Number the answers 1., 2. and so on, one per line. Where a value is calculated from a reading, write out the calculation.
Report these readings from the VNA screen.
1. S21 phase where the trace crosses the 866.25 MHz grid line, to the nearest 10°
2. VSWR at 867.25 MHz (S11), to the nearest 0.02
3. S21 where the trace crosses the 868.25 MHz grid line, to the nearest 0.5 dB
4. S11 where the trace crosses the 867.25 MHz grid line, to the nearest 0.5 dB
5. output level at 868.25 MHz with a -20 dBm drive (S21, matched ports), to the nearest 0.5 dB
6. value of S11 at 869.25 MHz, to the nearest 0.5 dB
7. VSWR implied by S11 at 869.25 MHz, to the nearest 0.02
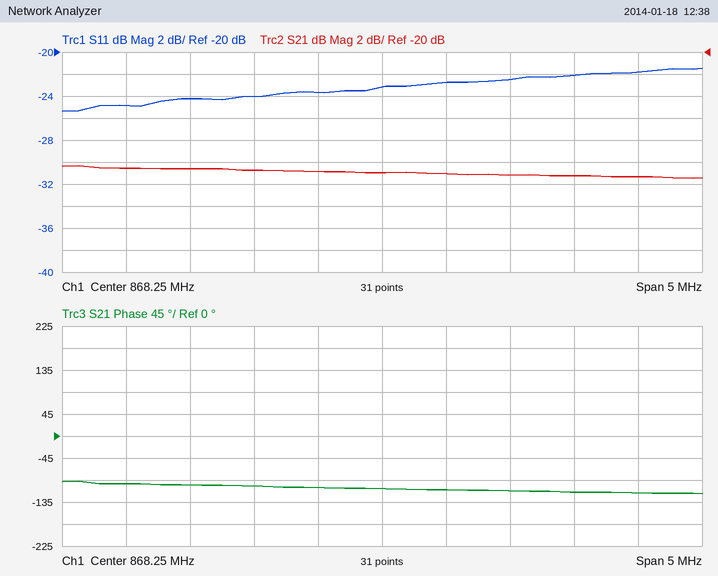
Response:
1. -100°
2. |Γ| = 10^(-24/20) = 0.0631; VSWR = (1 + 0.0631)/(1 − 0.0631) ≈ 1.13, so 1.14 to the nearest 0.02
3. -31.0 dB
4. -24.0 dB
5. -20 dBm + (-31.0 dB) = -51.0 dBm
6. -22.5 dB
7. |Γ| = 10^(-22.5/20) = 0.0750; VSWR = (1 + 0.0750)/(1 − 0.0750) ≈ 1.16
